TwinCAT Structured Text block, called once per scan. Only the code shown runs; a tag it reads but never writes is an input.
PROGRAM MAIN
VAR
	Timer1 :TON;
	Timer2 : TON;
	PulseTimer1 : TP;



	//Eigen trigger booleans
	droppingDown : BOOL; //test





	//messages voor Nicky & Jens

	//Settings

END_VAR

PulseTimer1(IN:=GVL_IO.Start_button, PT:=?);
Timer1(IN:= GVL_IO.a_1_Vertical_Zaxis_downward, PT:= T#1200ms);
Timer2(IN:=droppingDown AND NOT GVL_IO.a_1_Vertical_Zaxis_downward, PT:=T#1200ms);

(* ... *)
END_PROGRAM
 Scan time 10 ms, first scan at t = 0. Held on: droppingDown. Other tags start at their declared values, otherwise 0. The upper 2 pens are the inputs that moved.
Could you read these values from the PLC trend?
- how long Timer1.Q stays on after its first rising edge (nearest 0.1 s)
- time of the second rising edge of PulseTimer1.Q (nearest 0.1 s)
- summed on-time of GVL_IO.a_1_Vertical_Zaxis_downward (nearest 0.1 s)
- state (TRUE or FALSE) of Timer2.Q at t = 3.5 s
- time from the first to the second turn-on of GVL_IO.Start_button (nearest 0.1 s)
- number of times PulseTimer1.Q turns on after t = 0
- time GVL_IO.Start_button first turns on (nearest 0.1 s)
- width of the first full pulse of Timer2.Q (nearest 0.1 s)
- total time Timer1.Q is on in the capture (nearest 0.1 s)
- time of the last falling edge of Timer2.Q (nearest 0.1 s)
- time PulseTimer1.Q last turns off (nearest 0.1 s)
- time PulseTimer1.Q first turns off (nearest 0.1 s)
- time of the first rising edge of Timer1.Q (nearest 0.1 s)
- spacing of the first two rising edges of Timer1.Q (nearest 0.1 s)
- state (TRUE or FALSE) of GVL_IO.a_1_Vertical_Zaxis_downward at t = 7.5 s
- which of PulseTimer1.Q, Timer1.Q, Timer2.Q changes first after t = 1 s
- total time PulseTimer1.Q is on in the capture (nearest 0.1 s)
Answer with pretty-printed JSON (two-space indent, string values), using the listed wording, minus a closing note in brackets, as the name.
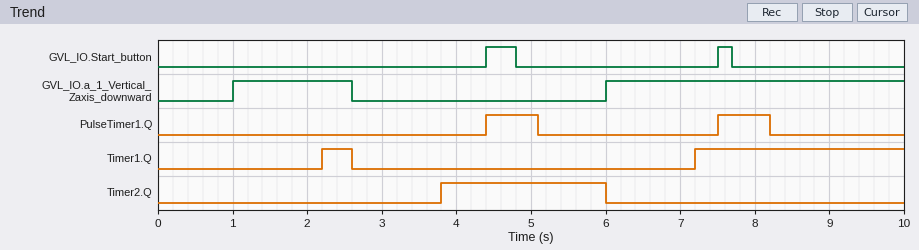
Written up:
{
  "how long Timer1.Q stays on after its first rising edge": "0.4 s",
  "time of the second rising edge of PulseTimer1.Q": "7.5 s",
  "summed on-time of GVL_IO.a_1_Vertical_Zaxis_downward": "5.6 s",
  "state (TRUE or FALSE) of Timer2.Q at t = 3.5 s": "FALSE",
  "time from the first to the second turn-on of GVL_IO.Start_button": "3.1 s",
  "number of times PulseTimer1.Q turns on after t = 0": "2",
  "time GVL_IO.Start_button first turns on": "4.4 s",
  "width of the first full pulse of Timer2.Q": "2.2 s",
  "total time Timer1.Q is on in the capture": "3.2 s",
  "time of the last falling edge of Timer2.Q": "6.0 s",
  "time PulseTimer1.Q last turns off": "8.2 s",
  "time PulseTimer1.Q first turns off": "5.1 s",
  "time of the first rising edge of Timer1.Q": "2.2 s",
  "spacing of the first two rising edges of Timer1.Q": "5.0 s",
  "state (TRUE or FALSE) of GVL_IO.a_1_Vertical_Zaxis_downward at t = 7.5 s": "TRUE",
  "which of PulseTimer1.Q, Timer1.Q, Timer2.Q changes first after t = 1 s": "Timer1.Q",
  "total time PulseTimer1.Q is on in the capture": "1.4 s"
}
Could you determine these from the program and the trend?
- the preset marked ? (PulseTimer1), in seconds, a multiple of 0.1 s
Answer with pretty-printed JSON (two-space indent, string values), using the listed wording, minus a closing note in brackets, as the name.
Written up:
{
  "the preset marked ? (PulseTimer1), in seconds, a multiple of 0.1 s": "0.7 s"
}
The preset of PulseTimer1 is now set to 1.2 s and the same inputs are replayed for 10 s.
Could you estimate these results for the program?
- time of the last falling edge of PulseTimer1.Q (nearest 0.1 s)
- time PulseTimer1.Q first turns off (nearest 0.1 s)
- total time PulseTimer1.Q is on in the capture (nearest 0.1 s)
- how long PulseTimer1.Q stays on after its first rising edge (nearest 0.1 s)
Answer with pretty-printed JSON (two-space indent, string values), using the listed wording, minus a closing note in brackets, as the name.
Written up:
{
  "time of the last falling edge of PulseTimer1.Q": "8.7 s",
  "time PulseTimer1.Q first turns off": "5.6 s",
  "total time PulseTimer1.Q is on in the capture": "2.4 s",
  "how long PulseTimer1.Q stays on after its first rising edge": "1.2 s"
}
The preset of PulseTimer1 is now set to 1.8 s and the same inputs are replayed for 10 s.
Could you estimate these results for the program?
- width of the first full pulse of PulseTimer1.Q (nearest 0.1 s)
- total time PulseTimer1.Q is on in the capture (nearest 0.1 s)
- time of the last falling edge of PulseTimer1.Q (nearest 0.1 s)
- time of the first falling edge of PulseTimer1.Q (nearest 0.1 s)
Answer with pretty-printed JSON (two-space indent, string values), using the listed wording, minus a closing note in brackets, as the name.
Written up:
{
  "width of the first full pulse of PulseTimer1.Q": "1.8 s",
  "total time PulseTimer1.Q is on in the capture": "3.6 s",
  "time of the last falling edge of PulseTimer1.Q": "9.3 s",
  "time of the first falling edge of PulseTimer1.Q": "6.2 s"
}
